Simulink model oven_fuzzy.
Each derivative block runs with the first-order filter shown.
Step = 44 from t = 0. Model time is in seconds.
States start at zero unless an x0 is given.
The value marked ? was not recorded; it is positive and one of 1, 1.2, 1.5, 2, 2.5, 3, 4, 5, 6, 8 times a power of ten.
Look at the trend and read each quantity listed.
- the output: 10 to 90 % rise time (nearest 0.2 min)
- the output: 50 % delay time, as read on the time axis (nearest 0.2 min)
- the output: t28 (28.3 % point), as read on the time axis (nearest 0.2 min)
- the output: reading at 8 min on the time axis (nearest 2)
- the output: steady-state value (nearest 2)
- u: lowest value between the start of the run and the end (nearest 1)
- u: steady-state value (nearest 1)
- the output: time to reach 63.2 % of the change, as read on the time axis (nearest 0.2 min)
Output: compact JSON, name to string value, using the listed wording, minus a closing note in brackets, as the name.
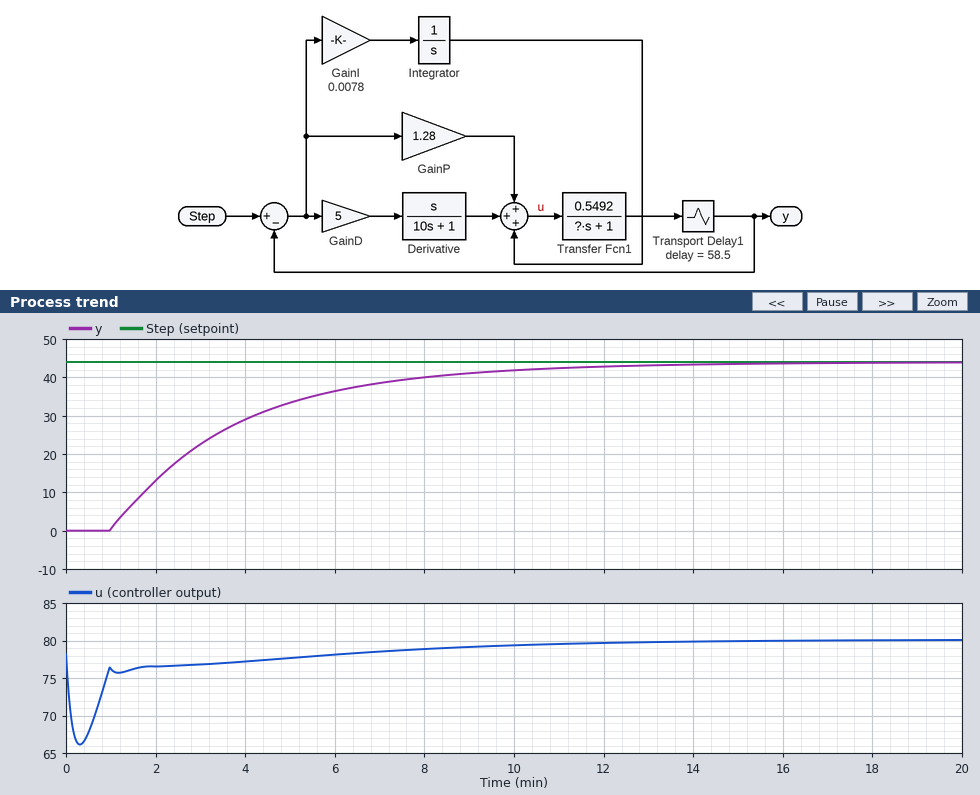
{"the output: 10 to 90 % rise time": "6.4 min", "the output: 50 % delay time, as read on the time axis": "3.0 min", "the output: t28 (28.3 % point), as read on the time axis": "2.0 min", "the output: reading at 8 min on the time axis": "40", "the output: steady-state value": "44", "u: lowest value between the start of the run and the end": "66", "u: steady-state value": "80", "the output: time to reach 63.2 % of the change, as read on the time axis": "3.8 min"}
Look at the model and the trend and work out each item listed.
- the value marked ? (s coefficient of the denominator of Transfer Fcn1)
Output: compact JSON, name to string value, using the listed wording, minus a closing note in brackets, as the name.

{"the value marked ?": "150"}
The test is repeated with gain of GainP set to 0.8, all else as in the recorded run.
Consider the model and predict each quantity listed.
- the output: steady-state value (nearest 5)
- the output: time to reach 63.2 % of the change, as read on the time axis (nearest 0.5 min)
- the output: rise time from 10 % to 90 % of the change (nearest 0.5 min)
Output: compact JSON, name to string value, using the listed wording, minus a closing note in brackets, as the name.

{"the output: steady-state value": "45", "the output: time to reach 63.2 % of the change, as read on the time axis": "4.5 min", "the output: rise time from 10 % to 90 % of the change": "6.0 min"}
